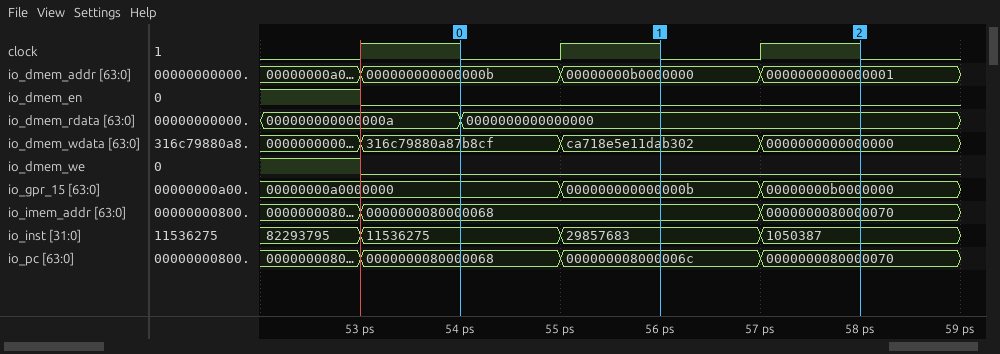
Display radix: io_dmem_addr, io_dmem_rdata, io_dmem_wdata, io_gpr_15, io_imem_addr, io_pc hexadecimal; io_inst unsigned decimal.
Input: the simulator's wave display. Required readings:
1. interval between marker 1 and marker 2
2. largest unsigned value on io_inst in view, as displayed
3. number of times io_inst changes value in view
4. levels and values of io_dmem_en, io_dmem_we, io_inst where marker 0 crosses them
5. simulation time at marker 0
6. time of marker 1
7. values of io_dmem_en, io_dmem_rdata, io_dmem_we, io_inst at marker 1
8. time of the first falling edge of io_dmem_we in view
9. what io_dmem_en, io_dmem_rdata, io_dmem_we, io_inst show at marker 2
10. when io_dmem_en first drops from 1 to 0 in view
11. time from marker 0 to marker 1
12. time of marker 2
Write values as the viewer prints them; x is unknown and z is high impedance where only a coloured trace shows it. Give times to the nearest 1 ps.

2 ps
82293795
3
io_dmem_en=0, io_dmem_we=0, io_inst=11536275
54 ps
56 ps
io_dmem_en=0, io_dmem_rdata=0000000000000000, io_dmem_we=0, io_inst=29857683
53 ps
io_dmem_en=0, io_dmem_rdata=0000000000000000, io_dmem_we=0, io_inst=1050387
53 ps
2 ps
58 ps
